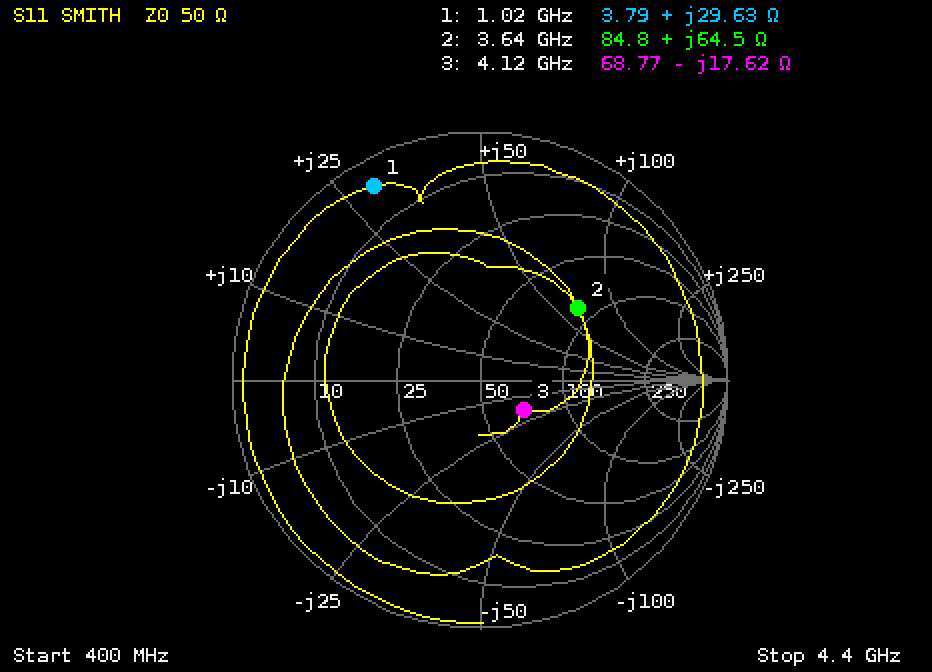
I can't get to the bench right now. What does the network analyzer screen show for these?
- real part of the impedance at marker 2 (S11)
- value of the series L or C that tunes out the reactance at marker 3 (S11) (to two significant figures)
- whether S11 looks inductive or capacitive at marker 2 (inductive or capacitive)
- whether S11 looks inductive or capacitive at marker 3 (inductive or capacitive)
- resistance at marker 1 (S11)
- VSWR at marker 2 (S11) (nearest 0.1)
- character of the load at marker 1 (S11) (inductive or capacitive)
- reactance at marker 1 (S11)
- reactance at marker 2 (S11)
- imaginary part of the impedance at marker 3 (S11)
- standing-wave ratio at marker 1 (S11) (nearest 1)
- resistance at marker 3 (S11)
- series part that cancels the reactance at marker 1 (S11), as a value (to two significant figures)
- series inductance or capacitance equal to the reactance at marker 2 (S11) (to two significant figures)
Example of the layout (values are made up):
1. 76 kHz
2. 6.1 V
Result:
1. 84.8 Ω
2. 680 pH
3. inductive
4. capacitive
5. 3.79 Ω
6. 2.9
7. inductive
8. +29.63 Ω
9. +64.5 Ω
10. -17.62 Ω
11. 18
12. 68.77 Ω
13. 5.3 pF
14. 2.8 nH
